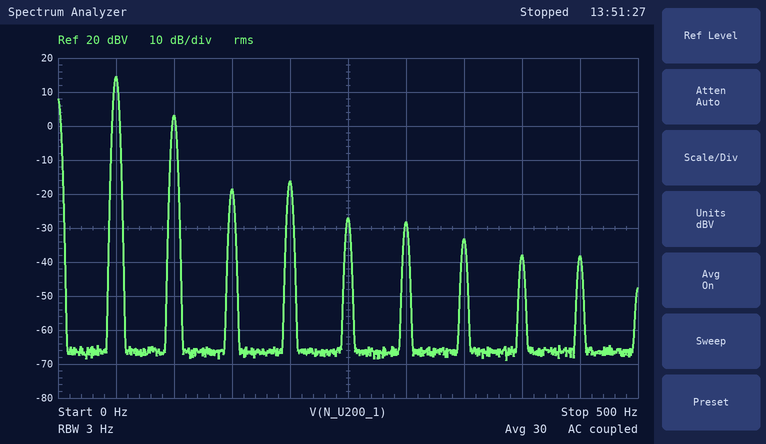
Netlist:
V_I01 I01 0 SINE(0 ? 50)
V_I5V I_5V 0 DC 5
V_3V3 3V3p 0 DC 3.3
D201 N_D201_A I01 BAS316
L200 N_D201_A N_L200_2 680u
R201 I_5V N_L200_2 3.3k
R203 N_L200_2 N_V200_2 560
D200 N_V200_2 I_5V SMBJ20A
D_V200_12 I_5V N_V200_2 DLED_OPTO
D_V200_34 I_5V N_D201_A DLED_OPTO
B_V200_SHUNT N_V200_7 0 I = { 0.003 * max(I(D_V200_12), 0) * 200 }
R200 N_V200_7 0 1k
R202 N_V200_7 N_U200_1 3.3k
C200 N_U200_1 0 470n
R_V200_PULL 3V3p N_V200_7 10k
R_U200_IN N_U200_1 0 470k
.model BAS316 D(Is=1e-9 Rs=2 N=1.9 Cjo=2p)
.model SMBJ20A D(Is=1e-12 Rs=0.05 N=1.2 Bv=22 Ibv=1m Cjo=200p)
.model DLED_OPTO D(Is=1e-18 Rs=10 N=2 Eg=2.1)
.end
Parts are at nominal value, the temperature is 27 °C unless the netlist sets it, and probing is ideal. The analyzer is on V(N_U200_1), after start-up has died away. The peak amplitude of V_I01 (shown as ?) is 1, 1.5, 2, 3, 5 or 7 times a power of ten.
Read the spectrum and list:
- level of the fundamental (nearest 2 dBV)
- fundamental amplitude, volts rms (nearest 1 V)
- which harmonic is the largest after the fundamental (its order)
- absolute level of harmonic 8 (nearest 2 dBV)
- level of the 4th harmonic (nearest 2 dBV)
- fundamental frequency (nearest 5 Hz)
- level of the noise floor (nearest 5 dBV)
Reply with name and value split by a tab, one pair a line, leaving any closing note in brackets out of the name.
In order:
level of the fundamental	14 dBV
fundamental amplitude, volts rms	5 V
which harmonic is the largest after the fundamental	2
absolute level of harmonic 8	-38 dBV
level of the 4th harmonic	-16 dBV
fundamental frequency	50 Hz
level of the noise floor	-65 dBV
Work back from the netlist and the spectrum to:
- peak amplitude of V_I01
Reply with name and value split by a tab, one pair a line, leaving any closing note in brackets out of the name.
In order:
peak amplitude of V_I01	20 V
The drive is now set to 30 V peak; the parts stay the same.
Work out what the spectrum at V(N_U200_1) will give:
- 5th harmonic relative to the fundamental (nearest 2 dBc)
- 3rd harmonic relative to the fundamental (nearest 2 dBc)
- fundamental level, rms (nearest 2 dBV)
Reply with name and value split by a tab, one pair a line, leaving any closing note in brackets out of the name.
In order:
5th harmonic relative to the fundamental	-44 dBc
3rd harmonic relative to the fundamental	-36 dBc
fundamental level, rms	18 dBV
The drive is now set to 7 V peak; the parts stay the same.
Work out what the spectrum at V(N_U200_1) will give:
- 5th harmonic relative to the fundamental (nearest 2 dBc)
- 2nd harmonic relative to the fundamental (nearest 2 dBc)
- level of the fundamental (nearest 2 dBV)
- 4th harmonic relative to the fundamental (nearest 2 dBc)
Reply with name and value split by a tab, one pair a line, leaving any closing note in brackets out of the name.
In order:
5th harmonic relative to the fundamental	-38 dBc
2nd harmonic relative to the fundamental	-14 dBc
level of the fundamental	8 dBV
4th harmonic relative to the fundamental	-44 dBc
